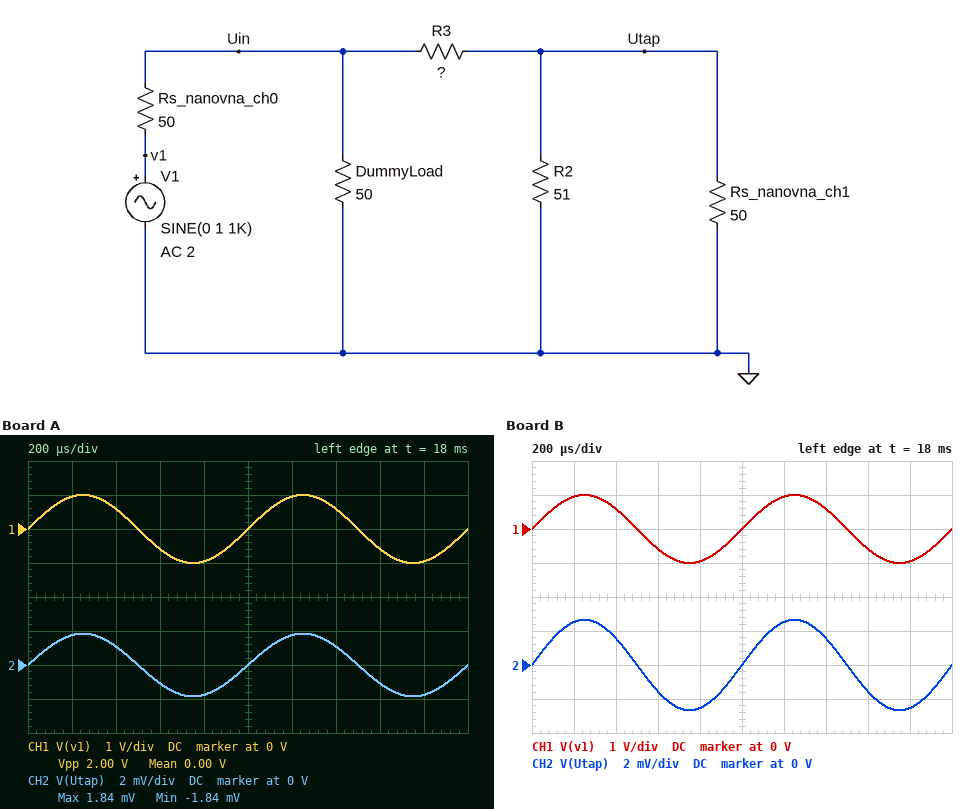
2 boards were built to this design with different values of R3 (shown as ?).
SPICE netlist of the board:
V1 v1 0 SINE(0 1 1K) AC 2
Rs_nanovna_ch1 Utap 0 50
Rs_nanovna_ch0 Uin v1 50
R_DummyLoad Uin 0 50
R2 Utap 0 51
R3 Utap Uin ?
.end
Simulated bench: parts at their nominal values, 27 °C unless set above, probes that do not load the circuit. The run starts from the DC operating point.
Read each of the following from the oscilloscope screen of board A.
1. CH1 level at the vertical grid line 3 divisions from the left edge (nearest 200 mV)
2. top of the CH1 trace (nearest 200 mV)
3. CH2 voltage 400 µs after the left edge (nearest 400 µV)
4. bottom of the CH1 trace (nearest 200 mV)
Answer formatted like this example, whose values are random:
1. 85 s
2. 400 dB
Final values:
1. -600 mV
2. 1.0 V
3. 1.2 mV
4. -1.0 V
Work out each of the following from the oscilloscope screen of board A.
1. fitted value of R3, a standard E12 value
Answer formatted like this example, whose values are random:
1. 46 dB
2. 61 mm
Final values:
1. 6.8 kΩ
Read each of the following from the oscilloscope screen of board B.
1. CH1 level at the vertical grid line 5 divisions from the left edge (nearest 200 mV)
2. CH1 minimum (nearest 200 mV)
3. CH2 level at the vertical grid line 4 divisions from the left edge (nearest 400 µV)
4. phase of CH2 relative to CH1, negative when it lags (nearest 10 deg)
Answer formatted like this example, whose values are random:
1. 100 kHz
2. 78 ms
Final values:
1. 0 V
2. -1.0 V
3. -2.4 mV
4. 0 deg
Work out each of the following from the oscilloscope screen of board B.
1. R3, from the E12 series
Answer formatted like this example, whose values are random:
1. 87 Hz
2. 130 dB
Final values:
1. 4.7 kΩ
